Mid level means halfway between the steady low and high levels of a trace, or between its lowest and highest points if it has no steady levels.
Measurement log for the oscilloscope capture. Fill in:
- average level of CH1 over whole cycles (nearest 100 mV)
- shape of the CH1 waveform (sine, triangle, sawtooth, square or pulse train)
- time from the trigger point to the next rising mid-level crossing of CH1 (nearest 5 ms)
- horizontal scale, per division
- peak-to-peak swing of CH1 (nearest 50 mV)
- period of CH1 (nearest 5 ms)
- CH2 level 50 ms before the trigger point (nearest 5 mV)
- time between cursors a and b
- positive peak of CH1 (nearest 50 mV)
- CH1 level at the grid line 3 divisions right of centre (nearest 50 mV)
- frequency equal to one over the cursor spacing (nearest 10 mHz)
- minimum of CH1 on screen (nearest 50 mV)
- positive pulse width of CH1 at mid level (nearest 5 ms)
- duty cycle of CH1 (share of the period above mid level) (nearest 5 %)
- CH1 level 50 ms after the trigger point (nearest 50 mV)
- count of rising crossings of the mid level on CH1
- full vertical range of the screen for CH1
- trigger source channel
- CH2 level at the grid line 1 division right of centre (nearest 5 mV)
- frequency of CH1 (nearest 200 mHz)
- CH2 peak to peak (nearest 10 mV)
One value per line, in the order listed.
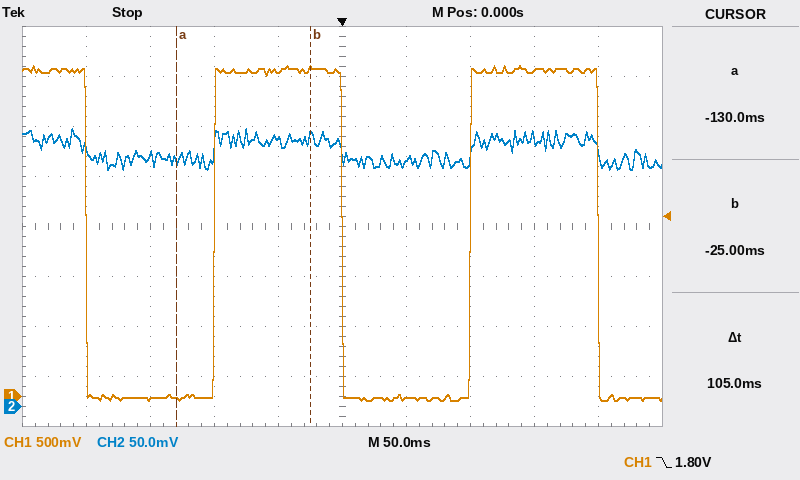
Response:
1.6 V
square
100 ms
50 ms
3.35 V
200 ms
265 mV
105 ms
3.30 V
3.25 V
9.52 Hz
-50 mV
100 ms
50 %
0 mV
2
4 V
CH1
245 mV
5.0 Hz
40 mV
